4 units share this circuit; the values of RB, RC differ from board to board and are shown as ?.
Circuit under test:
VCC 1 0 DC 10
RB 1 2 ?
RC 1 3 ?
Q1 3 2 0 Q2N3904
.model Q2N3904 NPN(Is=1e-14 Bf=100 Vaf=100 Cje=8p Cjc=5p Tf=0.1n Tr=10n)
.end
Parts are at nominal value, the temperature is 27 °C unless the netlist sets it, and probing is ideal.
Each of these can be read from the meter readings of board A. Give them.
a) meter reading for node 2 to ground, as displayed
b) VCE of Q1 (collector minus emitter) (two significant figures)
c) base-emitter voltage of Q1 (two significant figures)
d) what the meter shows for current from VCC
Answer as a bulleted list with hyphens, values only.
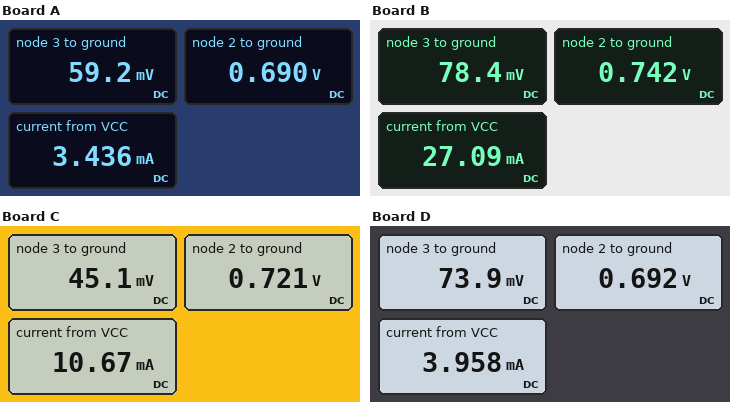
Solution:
- 0.690 V
- 59 mV
- 690 mV
- 3.436 mA
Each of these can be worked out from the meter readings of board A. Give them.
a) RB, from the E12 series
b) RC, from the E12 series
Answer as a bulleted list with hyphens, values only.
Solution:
- 22 kΩ
- 3.3 kΩ
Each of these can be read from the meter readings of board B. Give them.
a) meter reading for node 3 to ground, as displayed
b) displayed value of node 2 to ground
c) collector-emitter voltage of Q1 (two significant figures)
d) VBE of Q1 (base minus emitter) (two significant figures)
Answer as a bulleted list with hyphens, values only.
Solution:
- 78.4 mV
- 0.742 V
- 78 mV
- 740 mV
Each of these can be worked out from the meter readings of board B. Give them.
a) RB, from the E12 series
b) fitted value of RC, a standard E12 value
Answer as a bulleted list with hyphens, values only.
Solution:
- 5.6 kΩ
- 390 Ω
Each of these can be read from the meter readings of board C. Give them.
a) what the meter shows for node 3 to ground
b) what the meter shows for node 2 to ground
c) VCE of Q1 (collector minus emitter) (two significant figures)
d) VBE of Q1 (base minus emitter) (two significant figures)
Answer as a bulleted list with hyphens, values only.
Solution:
- 45.1 mV
- 0.721 V
- 45 mV
- 720 mV
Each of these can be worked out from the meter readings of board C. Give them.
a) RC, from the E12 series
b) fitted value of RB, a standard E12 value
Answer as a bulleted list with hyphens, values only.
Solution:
- 1.2 kΩ
- 3.9 kΩ
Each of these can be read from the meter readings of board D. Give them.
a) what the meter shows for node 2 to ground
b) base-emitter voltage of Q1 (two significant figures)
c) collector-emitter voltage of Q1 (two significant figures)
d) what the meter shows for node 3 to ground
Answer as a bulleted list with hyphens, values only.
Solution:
- 0.692 V
- 690 mV
- 74 mV
- 73.9 mV
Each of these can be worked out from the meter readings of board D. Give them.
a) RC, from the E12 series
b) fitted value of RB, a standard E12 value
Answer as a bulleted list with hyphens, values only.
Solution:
- 2.7 kΩ
- 33 kΩ
